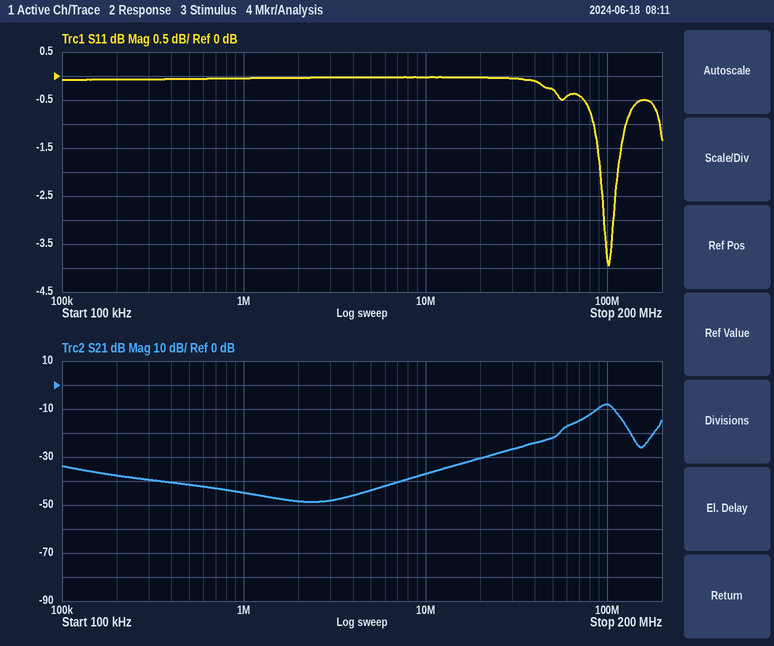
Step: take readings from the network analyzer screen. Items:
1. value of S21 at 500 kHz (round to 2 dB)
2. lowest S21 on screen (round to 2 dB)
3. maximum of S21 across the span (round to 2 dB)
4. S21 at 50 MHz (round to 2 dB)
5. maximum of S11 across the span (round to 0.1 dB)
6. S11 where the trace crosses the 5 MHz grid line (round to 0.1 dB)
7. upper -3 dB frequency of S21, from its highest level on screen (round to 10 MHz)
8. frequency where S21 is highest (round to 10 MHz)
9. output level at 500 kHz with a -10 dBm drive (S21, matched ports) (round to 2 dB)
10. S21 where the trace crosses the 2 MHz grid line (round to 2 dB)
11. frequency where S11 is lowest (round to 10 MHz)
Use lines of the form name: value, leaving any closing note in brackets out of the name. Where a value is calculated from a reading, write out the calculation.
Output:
value of S21 at 500 kHz: -42 dB
lowest S21 on screen: -48 dB
maximum of S21 across the span: -8 dB
S21 at 50 MHz: -22 dB
maximum of S11 across the span: 0.0 dB
S11 where the trace crosses the 5 MHz grid line: 0.0 dB
upper -3 dB frequency of S21, from its highest level on screen: 110 MHz
frequency where S21 is highest: 100 MHz
output level at 500 kHz with a -10 dBm drive (S21, matched ports): -10 dBm + (-42 dB) = -52 dBm
S21 where the trace crosses the 2 MHz grid line: -48 dB
frequency where S11 is lowest: 100 MHz
